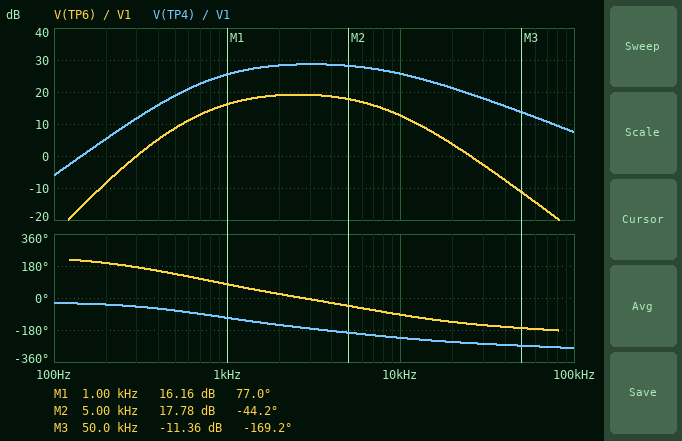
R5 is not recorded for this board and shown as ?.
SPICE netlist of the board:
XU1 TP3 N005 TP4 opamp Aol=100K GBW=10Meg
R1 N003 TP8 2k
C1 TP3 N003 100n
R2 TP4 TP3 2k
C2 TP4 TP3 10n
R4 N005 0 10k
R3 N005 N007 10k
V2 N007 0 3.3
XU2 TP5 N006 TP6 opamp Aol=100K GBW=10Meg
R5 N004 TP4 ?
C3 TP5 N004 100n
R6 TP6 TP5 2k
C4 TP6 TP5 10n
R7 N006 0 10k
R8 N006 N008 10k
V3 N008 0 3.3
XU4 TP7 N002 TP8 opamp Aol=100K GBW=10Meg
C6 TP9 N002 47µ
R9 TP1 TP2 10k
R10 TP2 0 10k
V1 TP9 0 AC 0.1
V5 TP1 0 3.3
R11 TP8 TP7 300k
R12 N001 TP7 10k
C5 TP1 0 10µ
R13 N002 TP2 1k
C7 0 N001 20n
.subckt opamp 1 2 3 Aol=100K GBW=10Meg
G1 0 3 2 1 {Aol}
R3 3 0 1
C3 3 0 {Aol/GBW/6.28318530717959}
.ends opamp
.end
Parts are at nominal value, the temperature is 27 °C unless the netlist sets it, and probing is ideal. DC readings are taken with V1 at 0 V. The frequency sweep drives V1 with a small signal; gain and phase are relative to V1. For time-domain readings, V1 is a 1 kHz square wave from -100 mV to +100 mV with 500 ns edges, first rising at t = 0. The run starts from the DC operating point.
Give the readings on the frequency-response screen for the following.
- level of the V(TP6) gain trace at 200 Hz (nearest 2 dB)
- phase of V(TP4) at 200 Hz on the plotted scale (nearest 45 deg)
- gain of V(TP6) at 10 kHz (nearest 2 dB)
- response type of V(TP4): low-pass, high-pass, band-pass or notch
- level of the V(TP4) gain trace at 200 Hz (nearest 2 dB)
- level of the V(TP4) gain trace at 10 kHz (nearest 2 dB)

-8 dB
-45 deg
12 dB
band-pass
6 dB
26 dB
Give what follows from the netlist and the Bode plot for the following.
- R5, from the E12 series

5.6 kΩ
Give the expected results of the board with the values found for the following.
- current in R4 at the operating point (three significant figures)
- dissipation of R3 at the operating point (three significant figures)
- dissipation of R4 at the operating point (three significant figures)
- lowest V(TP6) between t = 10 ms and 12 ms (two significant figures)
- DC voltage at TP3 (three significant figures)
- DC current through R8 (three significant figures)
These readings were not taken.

165 µA
272 µW
272 µW
160 mV
1.65 V
165 µA
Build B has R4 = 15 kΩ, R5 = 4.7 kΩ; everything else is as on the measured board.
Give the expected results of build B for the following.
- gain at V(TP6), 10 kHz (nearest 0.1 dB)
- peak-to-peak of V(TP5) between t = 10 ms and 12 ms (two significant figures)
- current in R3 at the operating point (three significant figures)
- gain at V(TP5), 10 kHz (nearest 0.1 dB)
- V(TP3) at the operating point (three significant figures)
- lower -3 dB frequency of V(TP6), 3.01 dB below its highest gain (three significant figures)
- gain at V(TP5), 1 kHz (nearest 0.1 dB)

14.1 dB
1.3 mV
132 µA
-45.9 dB
1.98 V
1.02 kHz
-62.4 dB
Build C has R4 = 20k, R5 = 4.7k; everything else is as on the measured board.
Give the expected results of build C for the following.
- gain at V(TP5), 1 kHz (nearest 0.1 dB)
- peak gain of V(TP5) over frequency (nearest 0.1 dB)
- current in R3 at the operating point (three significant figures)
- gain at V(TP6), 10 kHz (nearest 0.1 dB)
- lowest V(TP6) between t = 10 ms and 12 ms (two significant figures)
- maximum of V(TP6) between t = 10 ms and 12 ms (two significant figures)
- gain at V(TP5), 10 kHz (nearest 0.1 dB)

-62.4 dB
-45.7 dB
110 µA
14.1 dB
-110 mV
3.4 V
-45.9 dB
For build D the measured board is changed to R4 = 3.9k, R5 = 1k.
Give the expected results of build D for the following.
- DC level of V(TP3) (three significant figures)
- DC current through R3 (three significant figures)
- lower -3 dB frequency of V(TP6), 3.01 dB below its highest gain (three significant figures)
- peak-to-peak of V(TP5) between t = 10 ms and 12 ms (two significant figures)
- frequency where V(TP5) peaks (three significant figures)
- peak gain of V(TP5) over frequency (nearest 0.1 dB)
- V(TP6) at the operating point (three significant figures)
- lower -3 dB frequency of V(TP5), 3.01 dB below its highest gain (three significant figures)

926 mV
237 µA
1.49 kHz
5.6 mV
8.37 kHz
-32.4 dB
1.65 V
3.80 kHz
